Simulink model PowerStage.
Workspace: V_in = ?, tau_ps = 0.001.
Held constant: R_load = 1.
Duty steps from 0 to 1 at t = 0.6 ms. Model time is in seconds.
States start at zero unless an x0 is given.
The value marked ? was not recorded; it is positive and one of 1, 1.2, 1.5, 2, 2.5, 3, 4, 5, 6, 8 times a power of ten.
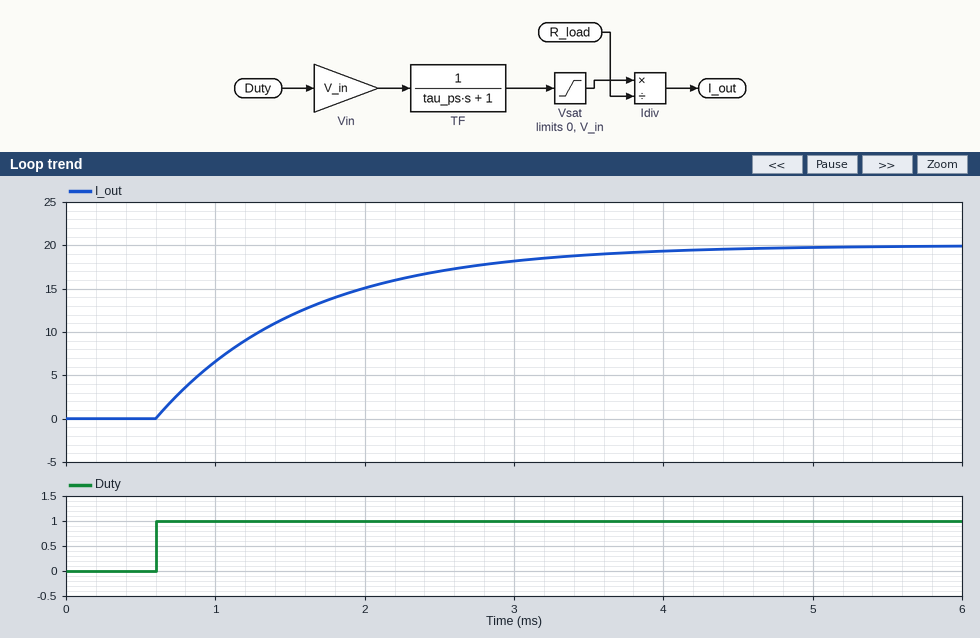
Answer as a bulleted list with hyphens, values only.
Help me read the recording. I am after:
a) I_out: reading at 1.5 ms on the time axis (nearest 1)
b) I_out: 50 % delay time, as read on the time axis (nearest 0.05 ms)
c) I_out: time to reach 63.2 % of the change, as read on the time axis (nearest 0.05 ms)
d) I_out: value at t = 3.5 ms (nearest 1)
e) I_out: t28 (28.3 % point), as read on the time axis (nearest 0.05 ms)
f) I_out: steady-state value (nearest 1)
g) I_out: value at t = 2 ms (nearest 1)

- 12
- 1.30 ms
- 1.60 ms
- 19
- 0.95 ms
- 20
- 15
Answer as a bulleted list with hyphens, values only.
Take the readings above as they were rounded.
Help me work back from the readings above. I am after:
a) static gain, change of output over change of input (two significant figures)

- 20
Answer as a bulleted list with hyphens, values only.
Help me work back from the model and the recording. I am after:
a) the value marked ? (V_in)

- 20
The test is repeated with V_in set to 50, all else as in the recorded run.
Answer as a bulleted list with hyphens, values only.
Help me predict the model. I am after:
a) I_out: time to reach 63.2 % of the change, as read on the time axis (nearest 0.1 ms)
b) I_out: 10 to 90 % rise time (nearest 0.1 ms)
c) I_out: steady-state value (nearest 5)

- 1.6 ms
- 2.2 ms
- 50
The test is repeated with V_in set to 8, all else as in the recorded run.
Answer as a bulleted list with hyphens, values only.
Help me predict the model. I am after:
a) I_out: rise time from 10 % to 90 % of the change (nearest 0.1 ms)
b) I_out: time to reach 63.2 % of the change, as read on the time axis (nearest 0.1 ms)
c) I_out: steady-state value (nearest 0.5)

- 2.2 ms
- 1.6 ms
- 8.0
